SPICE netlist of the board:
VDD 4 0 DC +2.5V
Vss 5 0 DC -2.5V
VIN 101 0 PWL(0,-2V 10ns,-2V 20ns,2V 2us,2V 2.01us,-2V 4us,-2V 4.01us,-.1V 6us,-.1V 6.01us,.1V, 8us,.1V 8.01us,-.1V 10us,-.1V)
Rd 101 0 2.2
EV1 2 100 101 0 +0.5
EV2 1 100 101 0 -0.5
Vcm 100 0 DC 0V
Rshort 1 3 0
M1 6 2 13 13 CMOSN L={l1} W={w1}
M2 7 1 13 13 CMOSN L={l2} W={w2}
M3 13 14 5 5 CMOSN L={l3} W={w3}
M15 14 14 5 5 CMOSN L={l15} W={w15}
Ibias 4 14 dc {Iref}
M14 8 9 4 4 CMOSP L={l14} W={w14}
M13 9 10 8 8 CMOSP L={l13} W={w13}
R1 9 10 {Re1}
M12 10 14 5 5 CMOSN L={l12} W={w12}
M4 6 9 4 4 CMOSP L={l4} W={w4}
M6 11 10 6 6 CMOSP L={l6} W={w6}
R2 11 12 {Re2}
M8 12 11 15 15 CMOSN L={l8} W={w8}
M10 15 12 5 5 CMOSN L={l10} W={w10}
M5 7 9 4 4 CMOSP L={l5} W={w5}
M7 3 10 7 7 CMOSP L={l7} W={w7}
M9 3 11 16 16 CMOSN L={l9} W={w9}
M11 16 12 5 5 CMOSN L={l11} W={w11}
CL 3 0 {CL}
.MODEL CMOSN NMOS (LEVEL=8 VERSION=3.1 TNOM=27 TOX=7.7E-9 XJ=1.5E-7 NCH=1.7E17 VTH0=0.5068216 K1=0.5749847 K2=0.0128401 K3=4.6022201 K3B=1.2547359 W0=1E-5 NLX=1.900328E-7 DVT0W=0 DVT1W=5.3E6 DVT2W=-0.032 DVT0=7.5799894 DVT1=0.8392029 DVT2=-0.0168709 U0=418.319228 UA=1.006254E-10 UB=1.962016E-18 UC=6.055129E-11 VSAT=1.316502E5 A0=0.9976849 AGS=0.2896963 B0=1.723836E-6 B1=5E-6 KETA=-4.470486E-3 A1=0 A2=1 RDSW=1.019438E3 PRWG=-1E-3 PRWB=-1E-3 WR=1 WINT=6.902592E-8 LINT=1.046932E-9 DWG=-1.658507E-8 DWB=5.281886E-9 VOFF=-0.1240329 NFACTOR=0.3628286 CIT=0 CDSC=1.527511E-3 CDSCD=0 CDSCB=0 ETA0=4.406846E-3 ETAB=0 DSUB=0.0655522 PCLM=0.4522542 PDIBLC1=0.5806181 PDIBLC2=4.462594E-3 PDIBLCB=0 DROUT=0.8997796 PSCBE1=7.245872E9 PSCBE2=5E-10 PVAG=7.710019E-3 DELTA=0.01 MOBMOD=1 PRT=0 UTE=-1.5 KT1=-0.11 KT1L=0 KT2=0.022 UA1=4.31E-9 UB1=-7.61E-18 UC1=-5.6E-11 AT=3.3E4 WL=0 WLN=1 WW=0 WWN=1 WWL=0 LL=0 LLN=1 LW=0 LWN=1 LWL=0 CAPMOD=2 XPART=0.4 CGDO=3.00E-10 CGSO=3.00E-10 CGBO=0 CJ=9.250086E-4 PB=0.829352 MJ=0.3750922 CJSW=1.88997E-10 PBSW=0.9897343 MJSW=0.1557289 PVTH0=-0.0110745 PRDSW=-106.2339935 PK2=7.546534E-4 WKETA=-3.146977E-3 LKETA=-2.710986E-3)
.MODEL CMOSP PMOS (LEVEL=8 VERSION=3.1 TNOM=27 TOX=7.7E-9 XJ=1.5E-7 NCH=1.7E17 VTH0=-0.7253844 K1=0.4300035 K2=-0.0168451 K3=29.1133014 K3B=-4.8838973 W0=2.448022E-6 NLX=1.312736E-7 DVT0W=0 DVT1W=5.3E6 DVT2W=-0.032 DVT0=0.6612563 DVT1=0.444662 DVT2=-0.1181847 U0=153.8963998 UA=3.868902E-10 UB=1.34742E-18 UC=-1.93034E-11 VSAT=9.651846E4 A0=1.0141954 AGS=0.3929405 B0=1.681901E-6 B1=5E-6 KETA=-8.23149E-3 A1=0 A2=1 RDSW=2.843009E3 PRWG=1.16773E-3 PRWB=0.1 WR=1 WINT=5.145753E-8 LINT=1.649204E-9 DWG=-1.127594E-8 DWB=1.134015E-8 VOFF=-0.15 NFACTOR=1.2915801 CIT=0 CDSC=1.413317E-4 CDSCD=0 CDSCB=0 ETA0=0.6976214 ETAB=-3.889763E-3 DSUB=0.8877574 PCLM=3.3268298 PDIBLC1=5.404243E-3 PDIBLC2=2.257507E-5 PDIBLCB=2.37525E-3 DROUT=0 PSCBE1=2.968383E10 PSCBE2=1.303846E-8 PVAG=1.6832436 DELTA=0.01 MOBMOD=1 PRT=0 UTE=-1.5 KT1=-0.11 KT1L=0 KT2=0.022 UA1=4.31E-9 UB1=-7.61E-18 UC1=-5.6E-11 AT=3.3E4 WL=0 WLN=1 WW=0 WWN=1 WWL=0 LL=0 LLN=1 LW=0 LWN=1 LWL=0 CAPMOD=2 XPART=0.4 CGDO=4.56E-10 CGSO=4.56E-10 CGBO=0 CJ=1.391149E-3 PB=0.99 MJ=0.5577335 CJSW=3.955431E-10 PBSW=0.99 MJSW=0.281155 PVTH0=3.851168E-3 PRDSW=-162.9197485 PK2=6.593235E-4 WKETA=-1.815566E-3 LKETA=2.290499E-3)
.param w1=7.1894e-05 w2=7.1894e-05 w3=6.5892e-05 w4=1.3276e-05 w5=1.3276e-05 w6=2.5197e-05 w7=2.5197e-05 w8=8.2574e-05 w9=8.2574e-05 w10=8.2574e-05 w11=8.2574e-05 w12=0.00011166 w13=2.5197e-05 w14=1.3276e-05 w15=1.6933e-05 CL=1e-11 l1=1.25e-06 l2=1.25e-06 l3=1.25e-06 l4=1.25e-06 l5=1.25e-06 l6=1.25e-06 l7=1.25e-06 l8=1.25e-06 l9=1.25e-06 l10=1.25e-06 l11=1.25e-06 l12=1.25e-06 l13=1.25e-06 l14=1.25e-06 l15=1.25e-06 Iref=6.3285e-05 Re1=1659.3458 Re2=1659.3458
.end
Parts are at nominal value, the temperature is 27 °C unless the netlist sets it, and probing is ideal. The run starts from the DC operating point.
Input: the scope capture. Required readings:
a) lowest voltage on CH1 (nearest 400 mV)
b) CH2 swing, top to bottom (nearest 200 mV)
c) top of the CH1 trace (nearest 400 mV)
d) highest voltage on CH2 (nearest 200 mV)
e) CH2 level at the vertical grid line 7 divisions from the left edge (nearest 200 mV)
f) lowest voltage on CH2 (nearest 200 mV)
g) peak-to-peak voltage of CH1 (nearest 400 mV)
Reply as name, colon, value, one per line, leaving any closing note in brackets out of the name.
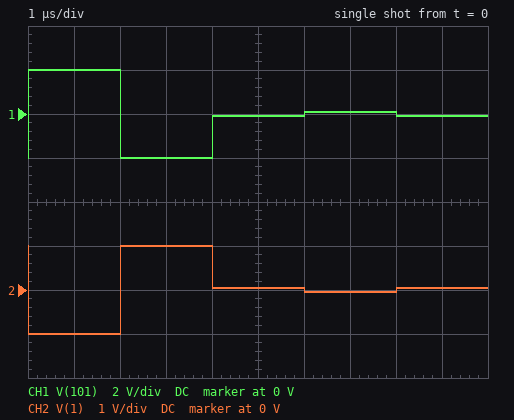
lowest voltage on CH1: -2.0 V
CH2 swing, top to bottom: 2.0 V
top of the CH1 trace: 2.0 V
highest voltage on CH2: 1.0 V
CH2 level at the vertical grid line 7 divisions from the left edge: 0 V
lowest voltage on CH2: -1.0 V
peak-to-peak voltage of CH1: 4.0 V
